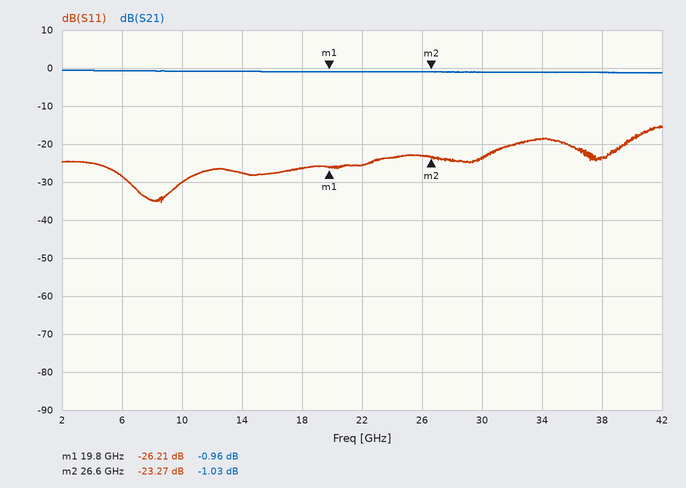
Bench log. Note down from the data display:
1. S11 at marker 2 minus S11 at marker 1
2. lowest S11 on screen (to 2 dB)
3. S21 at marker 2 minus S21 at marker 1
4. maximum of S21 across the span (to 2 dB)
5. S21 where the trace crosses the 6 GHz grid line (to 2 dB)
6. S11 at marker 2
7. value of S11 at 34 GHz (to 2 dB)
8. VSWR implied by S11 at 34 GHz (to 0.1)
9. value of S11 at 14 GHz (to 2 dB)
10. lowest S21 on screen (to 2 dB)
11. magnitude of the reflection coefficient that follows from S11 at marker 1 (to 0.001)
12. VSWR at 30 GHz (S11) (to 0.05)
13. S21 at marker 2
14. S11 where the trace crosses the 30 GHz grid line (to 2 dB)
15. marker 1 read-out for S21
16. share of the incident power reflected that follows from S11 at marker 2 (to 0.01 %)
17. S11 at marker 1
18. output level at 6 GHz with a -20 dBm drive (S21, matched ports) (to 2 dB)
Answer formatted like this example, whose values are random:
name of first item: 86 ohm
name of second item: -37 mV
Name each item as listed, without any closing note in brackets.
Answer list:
S11 at marker 2 minus S11 at marker 1: 2.94 dB
lowest S11 on screen: -36 dB
S21 at marker 2 minus S21 at marker 1: -0.07 dB
maximum of S21 across the span: 0 dB
S21 where the trace crosses the 6 GHz grid line: 0 dB
S11 at marker 2: -23.27 dB
value of S11 at 34 GHz: -18 dB
VSWR implied by S11 at 34 GHz: 1.3
value of S11 at 14 GHz: -28 dB
lowest S21 on screen: -2 dB
magnitude of the reflection coefficient that follows from S11 at marker 1: 0.049
VSWR at 30 GHz (S11): 1.15
S21 at marker 2: -1.03 dB
S11 where the trace crosses the 30 GHz grid line: -24 dB
marker 1 read-out for S21: -0.96 dB
share of the incident power reflected that follows from S11 at marker 2: 0.47 %
S11 at marker 1: -26.21 dB
output level at 6 GHz with a -20 dBm drive (S21, matched ports): -20 dBm
